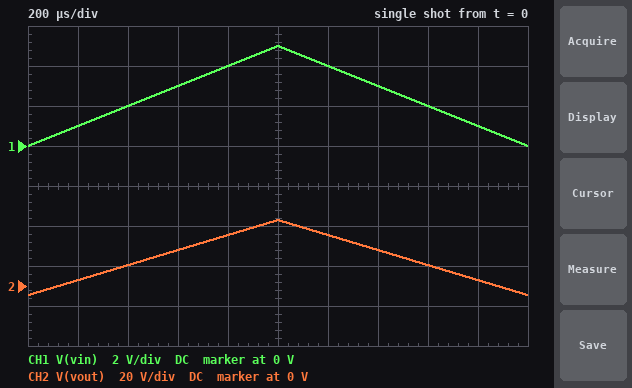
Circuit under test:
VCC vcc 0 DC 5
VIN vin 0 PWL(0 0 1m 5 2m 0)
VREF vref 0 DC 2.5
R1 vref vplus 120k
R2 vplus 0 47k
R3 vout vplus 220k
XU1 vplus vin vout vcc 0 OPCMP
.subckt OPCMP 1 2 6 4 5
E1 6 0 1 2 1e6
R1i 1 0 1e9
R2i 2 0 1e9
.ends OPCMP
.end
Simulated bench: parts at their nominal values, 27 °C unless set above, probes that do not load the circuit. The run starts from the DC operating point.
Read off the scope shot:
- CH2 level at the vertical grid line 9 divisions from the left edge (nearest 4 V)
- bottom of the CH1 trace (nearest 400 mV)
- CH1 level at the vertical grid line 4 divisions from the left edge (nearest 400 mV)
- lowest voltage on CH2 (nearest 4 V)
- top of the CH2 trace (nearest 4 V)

4 V
0 V
4.0 V
-4 V
32 V
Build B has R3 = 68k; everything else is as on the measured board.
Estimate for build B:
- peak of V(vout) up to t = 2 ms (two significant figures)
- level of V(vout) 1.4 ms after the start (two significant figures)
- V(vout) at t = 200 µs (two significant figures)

14 V
7.6 V
1.6 V
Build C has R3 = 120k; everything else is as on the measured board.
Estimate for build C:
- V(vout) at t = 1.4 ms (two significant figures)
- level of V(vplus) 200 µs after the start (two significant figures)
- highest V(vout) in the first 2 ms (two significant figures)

11 V
1.0 V
20 V
